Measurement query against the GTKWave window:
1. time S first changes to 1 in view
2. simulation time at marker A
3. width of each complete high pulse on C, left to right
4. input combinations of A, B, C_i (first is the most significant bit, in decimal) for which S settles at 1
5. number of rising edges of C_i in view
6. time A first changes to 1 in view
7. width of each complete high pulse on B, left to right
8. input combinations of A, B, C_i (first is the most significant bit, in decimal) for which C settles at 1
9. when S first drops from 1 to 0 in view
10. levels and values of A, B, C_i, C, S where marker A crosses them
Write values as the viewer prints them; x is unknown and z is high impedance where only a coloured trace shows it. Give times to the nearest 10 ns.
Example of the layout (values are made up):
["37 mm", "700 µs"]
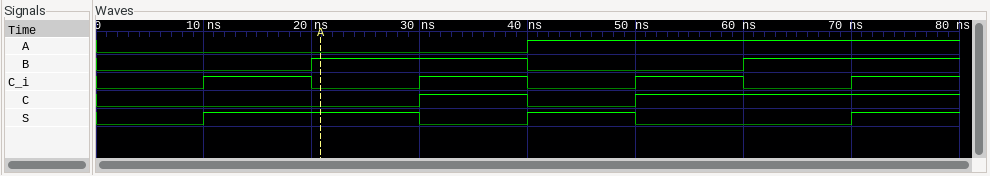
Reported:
["10 ns", "20 ns", "10 ns", "1, 2, 4, 7", "4", "40 ns", "20 ns", "3, 5, 6, 7", "30 ns", "A=0, B=1, C_i=0, C=0, S=1"]
